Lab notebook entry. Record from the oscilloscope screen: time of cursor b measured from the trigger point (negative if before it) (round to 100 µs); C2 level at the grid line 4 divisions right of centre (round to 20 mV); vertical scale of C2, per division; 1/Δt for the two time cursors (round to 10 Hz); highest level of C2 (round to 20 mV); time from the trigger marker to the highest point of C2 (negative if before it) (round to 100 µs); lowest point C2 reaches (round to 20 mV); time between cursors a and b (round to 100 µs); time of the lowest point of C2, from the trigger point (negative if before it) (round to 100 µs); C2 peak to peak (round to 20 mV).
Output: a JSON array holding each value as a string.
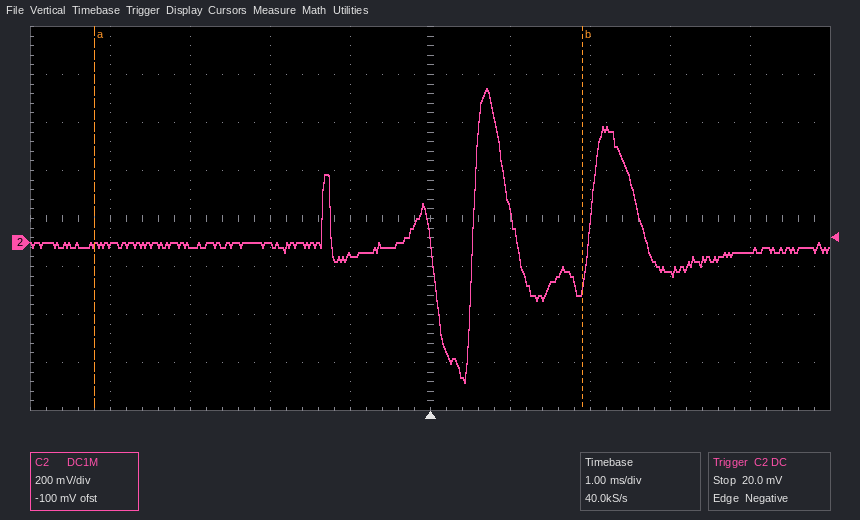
["+1.9 ms", "-40 mV", "200 mV", "160 Hz", "640 mV", "+700 µs", "-580 mV", "6.1 ms", "+400 µs", "1.22 V"]
